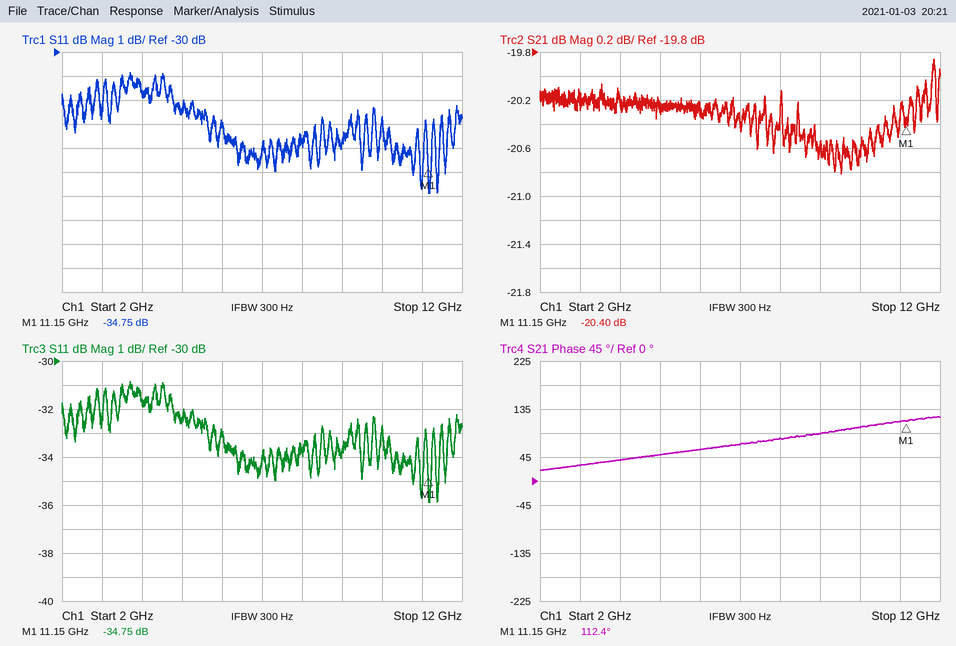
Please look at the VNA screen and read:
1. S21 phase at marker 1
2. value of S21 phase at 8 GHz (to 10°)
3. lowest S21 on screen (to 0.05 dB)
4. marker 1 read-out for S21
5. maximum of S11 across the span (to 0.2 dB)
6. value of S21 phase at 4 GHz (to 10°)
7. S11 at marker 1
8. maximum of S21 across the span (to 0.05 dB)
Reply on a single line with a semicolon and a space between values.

112.4°; 80°; -20.80 dB; -20.40 dB; -30.8 dB; 40°; -34.75 dB; -19.85 dB
